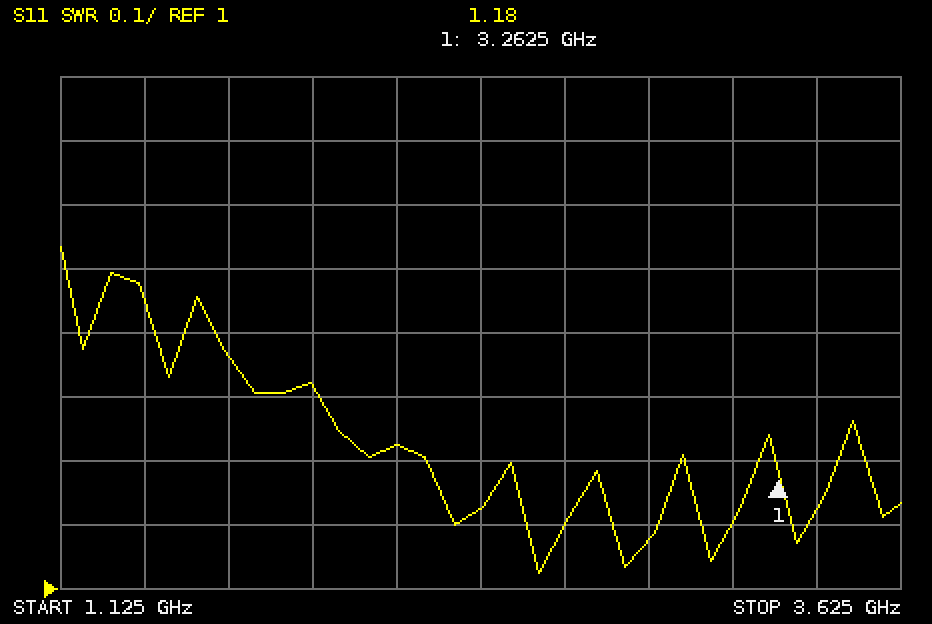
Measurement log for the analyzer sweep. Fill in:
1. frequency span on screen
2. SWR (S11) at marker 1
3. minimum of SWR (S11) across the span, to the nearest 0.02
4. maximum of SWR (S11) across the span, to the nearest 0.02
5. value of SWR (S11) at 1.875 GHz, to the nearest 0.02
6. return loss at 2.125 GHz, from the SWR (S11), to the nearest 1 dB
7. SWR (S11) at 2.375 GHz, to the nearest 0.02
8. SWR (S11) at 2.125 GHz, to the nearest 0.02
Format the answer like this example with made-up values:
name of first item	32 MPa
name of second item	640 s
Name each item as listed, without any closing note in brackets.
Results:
frequency span on screen	2.5 GHz
SWR (S11) at marker 1	1.18
minimum of SWR (S11) across the span, to the nearest 0.02	1.02
maximum of SWR (S11) across the span, to the nearest 0.02	1.54
value of SWR (S11) at 1.875 GHz, to the nearest 0.02	1.32
return loss at 2.125 GHz, from the SWR (S11), to the nearest 1 dB	20 dB
SWR (S11) at 2.375 GHz, to the nearest 0.02	1.12
SWR (S11) at 2.125 GHz, to the nearest 0.02	1.22
